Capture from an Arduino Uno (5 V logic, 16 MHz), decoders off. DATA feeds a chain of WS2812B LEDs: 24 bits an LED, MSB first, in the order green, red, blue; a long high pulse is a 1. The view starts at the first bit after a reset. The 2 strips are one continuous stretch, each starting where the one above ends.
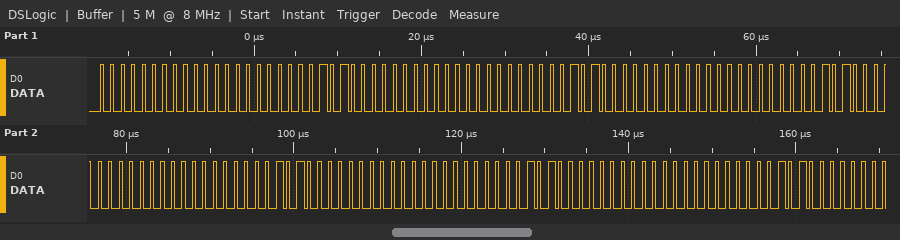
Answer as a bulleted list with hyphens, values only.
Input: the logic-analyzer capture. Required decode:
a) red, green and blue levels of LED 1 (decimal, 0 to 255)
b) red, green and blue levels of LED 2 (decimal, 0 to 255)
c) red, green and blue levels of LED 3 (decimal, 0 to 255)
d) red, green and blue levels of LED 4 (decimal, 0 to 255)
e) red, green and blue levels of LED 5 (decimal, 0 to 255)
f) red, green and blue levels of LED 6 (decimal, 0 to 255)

- 0, 0, 5
- 0, 0, 5
- 0, 0, 5
- 0, 0, 5
- 0, 0, 5
- 0, 0, 5
